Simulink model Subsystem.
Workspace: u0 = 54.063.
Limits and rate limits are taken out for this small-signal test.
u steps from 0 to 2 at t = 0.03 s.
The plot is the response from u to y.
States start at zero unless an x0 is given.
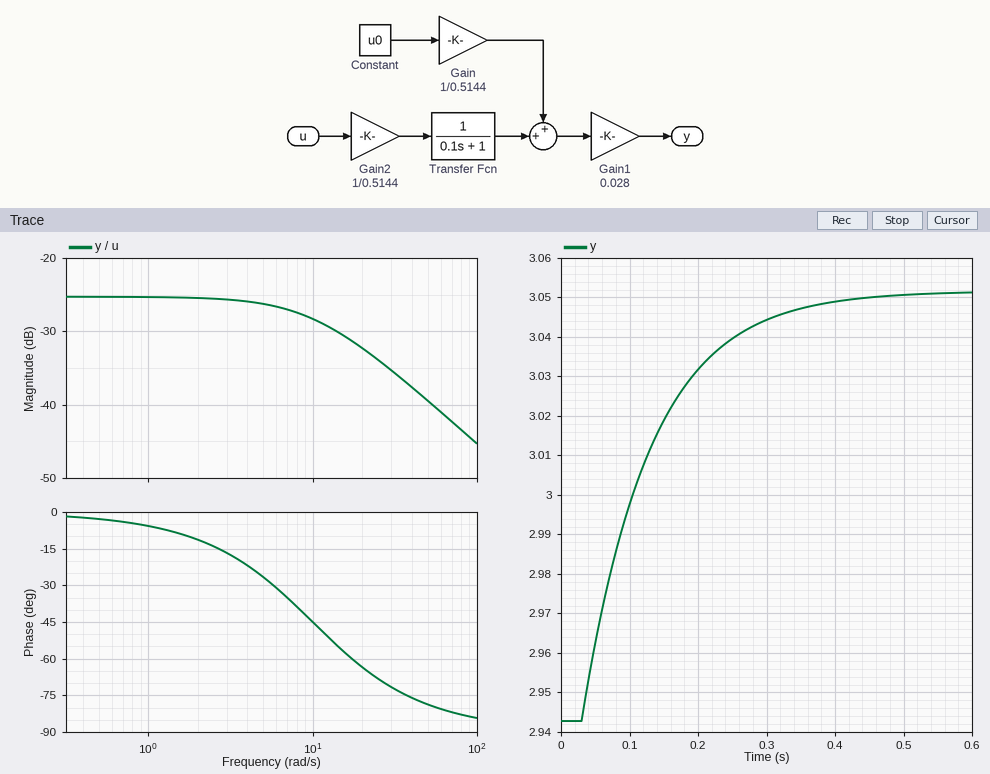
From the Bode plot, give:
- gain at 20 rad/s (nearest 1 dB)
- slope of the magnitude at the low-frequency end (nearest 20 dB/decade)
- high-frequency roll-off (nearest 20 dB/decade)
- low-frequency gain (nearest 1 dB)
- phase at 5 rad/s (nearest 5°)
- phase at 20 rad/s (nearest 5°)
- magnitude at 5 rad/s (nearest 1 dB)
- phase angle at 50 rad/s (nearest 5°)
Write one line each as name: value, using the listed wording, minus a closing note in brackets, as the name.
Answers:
gain at 20 rad/s: -32 dB
slope of the magnitude at the low-frequency end: 0 dB/decade
high-frequency roll-off: -20 dB/decade
low-frequency gain: -25 dB
phase at 5 rad/s: -25°
phase at 20 rad/s: -65°
magnitude at 5 rad/s: -26 dB
phase angle at 50 rad/s: -80°
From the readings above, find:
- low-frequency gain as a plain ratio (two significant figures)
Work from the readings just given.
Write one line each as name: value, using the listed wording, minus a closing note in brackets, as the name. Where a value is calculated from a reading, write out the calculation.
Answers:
low-frequency gain as a plain ratio: 10^(-25 / 20) = 0.056
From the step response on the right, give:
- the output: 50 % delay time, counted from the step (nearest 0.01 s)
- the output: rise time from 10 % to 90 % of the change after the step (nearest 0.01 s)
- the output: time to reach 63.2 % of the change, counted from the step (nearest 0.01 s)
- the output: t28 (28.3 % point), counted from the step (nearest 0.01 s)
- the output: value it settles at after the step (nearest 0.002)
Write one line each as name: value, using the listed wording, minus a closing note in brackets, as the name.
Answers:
the output: 50 % delay time, counted from the step: 0.07 s
the output: rise time from 10 % to 90 % of the change after the step: 0.22 s
the output: time to reach 63.2 % of the change, counted from the step: 0.10 s
the output: t28 (28.3 % point), counted from the step: 0.03 s
the output: value it settles at after the step: 3.052
